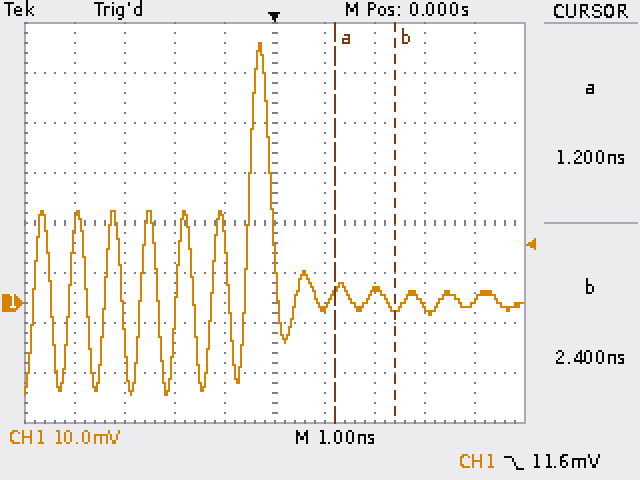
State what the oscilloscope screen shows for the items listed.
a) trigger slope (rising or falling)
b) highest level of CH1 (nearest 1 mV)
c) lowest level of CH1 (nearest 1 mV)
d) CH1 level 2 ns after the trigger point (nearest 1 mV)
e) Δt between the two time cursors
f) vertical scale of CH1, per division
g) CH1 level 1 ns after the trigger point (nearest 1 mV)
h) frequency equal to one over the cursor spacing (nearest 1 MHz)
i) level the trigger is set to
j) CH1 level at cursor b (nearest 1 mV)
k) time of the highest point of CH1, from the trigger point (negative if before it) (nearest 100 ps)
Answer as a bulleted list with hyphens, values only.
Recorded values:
- falling
- 52 mV
- -18 mV
- 2 mV
- 1.2 ns
- 10 mV
- -1 mV
- 833 MHz
- 11.6 mV
- -1 mV
- -300 ps
